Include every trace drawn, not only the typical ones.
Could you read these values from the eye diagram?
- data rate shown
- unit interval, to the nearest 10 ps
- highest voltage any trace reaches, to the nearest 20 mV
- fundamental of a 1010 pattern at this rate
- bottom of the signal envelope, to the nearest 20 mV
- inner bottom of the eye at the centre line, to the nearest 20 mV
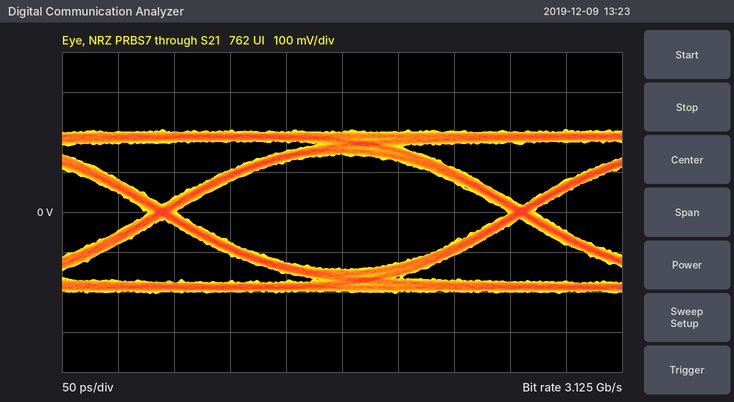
3.125 Gb/s
320 ps
200 mV
1.5625 GHz
-200 mV
-140 mV
